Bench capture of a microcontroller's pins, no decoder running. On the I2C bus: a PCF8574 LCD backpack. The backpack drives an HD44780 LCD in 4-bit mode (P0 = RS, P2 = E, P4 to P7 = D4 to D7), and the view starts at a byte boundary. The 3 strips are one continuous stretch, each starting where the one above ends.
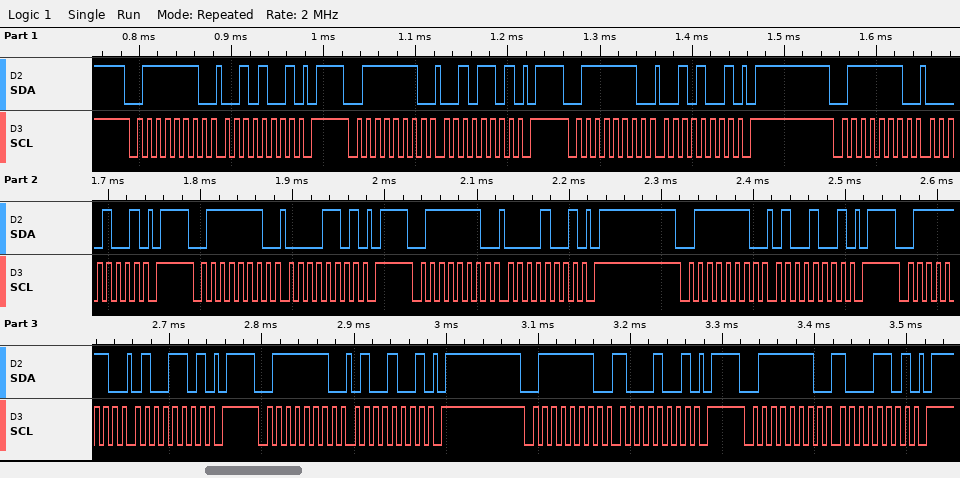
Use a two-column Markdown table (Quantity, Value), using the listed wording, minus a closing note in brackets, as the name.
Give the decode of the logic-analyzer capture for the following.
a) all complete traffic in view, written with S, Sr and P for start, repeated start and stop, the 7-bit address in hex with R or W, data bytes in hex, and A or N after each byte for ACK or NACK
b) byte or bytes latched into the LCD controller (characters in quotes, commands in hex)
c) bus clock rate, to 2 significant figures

| Quantity | Value |
|---|---|
| all complete traffic in view, written with S, Sr and P for start, repeated start and stop, the 7-bit address in hex with R or W, data bytes in hex, and A or N after each byte for ACK or NACK | S 3FW A 29 A P S 3FW A 2D A P S 3FW A 29 A P S 3FW A 09 A P S 3FW A 0D A P S 3FW A 09 A P S 3FW A 49 A P S 3FW A 4D A P S 3FW A 49 A P S 3FW A 89 A P S 3FW A 8D A P |
| byte or bytes latched into the LCD controller | ' ' |
| bus clock rate, to 2 significant figures | 100 kHz |
